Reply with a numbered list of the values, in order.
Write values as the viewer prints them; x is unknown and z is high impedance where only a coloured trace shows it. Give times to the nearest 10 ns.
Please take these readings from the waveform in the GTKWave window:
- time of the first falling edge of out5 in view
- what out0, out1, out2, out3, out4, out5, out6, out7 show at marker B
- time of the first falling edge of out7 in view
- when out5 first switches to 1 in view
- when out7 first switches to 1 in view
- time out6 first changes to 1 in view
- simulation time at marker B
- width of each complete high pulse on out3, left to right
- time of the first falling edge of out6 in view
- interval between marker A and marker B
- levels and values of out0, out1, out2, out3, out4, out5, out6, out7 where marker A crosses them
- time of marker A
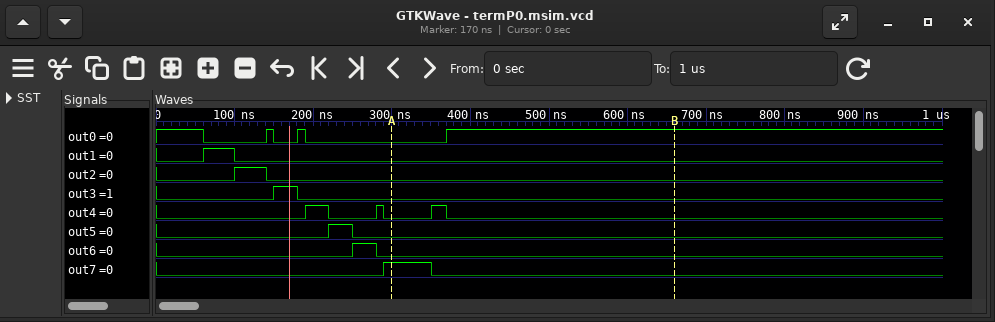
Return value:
1. 250 ns
2. out0=1, out1=0, out2=0, out3=0, out4=0, out5=0, out6=0, out7=0
3. 350 ns
4. 220 ns
5. 290 ns
6. 250 ns
7. 660 ns
8. 30 ns
9. 280 ns
10. 360 ns
11. out0=0, out1=0, out2=0, out3=0, out4=0, out5=0, out6=0, out7=1
12. 300 ns
